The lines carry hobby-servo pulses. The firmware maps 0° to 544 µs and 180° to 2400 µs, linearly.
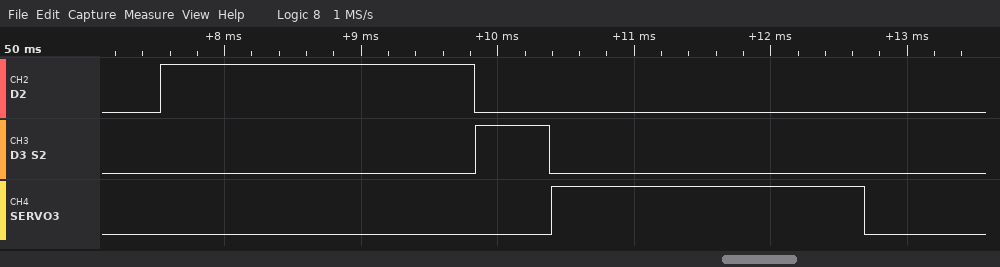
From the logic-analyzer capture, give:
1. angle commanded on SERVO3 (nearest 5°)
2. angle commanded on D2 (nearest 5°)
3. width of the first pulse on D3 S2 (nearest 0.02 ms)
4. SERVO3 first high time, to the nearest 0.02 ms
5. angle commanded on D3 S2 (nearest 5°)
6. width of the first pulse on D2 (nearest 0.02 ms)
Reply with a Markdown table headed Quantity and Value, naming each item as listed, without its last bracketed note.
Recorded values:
| Quantity | Value |
|---|---|
| angle commanded on SERVO3 | 170° |
| angle commanded on D2 | 170° |
| width of the first pulse on D3 S2 | 0.54 ms |
| SERVO3 first high time, to the nearest 0.02 ms | 2.30 ms |
| angle commanded on D3 S2 | 0° |
| width of the first pulse on D2 | 2.30 ms |
